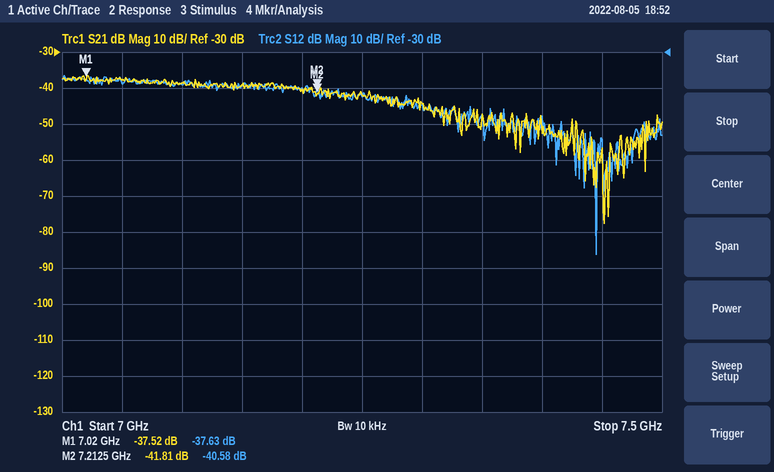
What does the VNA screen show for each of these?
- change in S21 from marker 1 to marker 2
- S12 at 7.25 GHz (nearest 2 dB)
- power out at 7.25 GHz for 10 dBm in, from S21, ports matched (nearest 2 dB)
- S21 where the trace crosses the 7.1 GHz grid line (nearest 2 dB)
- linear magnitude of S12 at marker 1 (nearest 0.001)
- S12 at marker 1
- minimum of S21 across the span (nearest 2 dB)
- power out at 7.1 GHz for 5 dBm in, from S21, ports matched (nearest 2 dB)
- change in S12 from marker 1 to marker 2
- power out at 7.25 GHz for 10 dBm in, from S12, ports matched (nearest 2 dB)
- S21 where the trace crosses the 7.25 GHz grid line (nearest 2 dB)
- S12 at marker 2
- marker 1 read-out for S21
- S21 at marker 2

-4.29 dB
-42 dB
-32 dBm
-38 dB
0.013
-37.63 dB
-78 dB
-34 dBm
-2.95 dB
-32 dBm
-42 dB
-40.58 dB
-37.52 dB
-41.81 dB
